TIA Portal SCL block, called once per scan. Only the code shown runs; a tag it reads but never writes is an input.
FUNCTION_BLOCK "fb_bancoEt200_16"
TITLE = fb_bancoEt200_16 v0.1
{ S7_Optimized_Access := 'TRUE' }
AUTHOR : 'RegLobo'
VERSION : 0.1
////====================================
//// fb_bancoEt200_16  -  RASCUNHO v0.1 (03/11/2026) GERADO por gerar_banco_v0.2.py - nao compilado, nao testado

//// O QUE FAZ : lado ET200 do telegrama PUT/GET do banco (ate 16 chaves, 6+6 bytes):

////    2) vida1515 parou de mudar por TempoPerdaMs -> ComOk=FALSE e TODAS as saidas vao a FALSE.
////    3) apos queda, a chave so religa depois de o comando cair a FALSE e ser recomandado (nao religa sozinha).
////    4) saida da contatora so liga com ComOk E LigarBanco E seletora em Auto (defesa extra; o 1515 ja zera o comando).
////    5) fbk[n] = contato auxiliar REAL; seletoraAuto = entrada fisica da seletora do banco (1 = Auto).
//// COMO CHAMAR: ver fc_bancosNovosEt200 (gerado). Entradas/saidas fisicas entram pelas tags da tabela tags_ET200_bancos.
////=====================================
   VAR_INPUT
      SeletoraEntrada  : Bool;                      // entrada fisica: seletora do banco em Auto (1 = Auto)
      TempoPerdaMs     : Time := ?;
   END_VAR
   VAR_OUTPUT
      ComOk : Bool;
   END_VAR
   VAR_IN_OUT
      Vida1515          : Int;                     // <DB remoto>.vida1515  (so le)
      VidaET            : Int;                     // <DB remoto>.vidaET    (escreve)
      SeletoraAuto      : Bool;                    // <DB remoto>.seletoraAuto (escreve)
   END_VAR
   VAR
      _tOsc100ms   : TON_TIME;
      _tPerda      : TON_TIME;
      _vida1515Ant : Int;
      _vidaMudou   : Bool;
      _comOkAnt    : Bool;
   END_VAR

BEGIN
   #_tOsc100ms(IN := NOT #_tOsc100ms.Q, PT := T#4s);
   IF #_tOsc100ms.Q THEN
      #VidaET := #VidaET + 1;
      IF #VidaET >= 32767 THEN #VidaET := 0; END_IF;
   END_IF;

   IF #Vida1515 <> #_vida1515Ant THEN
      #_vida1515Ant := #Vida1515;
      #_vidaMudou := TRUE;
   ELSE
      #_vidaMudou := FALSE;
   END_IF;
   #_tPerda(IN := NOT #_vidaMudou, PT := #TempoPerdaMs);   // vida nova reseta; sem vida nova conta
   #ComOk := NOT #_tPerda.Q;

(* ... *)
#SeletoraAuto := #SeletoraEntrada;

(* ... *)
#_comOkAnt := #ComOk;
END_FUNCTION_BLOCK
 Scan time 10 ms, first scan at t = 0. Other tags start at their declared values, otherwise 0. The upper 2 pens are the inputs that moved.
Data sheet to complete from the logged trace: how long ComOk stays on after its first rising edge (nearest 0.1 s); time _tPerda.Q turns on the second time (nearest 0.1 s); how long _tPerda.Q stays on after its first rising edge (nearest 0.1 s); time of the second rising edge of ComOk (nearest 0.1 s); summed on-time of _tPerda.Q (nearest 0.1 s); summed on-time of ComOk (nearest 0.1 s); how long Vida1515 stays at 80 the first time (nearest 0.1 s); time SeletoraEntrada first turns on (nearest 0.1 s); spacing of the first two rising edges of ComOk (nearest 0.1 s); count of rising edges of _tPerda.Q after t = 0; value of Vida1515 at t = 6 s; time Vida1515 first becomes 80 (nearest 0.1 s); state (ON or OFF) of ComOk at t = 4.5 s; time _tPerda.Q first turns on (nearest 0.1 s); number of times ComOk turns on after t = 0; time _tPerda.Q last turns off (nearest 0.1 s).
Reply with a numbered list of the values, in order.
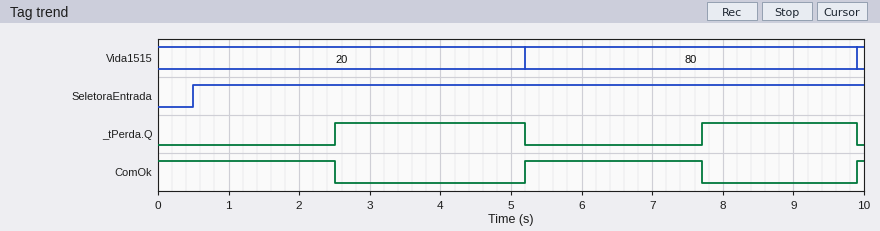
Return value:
1. 2.5 s
2. 7.7 s
3. 2.7 s
4. 9.9 s
5. 4.9 s
6. 5.1 s
7. 4.7 s
8. 0.5 s
9. 4.7 s
10. 2
11. 80
12. 5.2 s
13. OFF
14. 2.5 s
15. 2
16. 9.9 s
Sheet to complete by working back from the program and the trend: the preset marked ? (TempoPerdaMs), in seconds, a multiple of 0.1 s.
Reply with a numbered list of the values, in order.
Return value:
1. 2.5 s
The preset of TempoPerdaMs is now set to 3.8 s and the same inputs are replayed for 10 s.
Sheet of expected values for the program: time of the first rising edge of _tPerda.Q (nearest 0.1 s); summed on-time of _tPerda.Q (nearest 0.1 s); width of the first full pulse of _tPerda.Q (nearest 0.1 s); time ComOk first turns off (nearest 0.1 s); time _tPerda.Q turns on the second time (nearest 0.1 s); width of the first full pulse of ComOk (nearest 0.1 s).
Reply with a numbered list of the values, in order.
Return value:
1. 3.8 s
2. 2.3 s
3. 1.4 s
4. 3.8 s
5. 9.0 s
6. 3.8 s
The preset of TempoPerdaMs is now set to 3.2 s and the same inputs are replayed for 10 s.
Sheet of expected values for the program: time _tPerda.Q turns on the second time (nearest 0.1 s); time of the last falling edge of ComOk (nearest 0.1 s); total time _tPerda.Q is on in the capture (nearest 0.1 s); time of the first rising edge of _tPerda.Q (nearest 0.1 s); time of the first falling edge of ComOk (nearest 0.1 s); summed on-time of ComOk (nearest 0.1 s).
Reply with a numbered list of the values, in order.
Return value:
1. 8.4 s
2. 8.4 s
3. 3.5 s
4. 3.2 s
5. 3.2 s
6. 6.5 s
